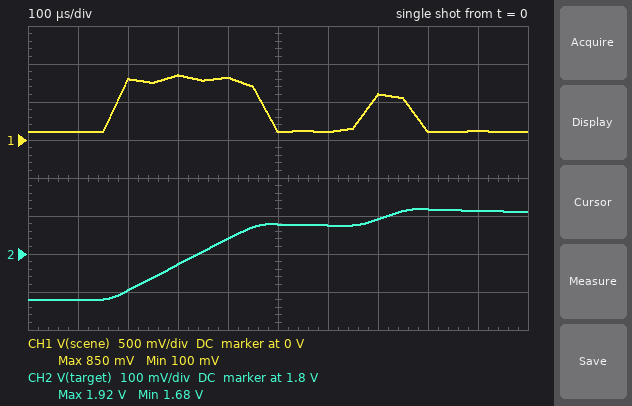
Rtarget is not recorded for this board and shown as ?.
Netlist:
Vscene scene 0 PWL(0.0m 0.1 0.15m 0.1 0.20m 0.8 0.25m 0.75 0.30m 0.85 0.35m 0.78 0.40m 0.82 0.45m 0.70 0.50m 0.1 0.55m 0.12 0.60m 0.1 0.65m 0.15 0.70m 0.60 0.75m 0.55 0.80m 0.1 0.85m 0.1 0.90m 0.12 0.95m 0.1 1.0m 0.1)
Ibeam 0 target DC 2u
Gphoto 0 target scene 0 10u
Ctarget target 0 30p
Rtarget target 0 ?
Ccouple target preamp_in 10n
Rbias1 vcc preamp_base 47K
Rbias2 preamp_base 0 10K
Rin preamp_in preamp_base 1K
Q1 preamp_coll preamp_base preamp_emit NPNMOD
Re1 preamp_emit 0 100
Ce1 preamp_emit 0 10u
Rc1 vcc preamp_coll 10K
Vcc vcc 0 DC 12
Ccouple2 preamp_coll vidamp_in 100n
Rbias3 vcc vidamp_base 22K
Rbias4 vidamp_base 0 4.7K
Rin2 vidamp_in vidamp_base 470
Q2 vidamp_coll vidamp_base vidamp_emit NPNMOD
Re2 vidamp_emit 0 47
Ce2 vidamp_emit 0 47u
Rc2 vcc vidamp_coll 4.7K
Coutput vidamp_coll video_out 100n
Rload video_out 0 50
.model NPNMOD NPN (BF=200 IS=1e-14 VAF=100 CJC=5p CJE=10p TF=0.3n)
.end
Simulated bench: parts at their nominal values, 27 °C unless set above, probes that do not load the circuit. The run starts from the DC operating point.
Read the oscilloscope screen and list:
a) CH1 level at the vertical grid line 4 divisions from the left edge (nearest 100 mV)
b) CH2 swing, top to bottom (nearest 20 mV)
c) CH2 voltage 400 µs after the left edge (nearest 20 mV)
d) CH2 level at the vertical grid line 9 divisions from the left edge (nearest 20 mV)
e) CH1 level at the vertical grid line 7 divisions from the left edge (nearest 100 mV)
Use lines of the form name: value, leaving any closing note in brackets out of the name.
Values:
CH1 level at the vertical grid line 4 divisions from the left edge: 800 mV
CH2 swing, top to bottom: 240 mV
CH2 voltage 400 µs after the left edge: 1.84 V
CH2 level at the vertical grid line 9 divisions from the left edge: 1.92 V
CH1 level at the vertical grid line 7 divisions from the left edge: 600 mV
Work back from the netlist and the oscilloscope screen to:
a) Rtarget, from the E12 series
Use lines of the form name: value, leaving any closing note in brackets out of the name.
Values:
Rtarget, from the E12 series: 560 kΩ
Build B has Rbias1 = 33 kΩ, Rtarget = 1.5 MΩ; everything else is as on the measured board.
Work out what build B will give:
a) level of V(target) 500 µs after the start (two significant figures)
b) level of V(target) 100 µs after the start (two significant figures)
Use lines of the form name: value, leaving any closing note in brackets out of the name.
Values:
level of V(target) 500 µs after the start: 4.7 V
level of V(target) 100 µs after the start: 4.5 V
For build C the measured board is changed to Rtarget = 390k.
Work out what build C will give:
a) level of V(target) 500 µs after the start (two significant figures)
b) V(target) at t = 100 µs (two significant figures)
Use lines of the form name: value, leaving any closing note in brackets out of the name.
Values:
level of V(target) 500 µs after the start: 1.4 V
V(target) at t = 100 µs: 1.2 V
